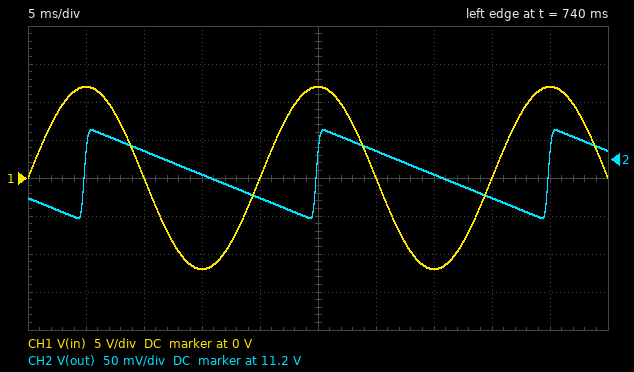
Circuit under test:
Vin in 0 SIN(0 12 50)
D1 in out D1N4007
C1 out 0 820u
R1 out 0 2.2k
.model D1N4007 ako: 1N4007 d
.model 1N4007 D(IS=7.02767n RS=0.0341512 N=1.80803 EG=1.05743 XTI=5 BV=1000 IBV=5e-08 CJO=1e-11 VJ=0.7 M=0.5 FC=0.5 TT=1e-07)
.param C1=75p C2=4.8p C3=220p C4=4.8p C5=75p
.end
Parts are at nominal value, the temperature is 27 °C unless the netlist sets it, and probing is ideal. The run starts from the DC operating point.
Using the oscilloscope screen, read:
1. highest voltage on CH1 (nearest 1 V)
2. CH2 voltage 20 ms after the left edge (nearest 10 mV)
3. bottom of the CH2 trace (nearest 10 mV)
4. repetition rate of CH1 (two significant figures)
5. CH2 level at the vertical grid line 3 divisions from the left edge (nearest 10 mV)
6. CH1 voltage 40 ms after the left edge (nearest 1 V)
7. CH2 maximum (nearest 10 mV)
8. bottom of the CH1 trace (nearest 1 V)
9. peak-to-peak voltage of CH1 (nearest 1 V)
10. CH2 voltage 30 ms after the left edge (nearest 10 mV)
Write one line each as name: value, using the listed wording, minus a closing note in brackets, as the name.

highest voltage on CH1: 12 V
CH2 voltage 20 ms after the left edge: 11.15 V
bottom of the CH2 trace: 11.12 V
repetition rate of CH1: 50 Hz
CH2 level at the vertical grid line 3 divisions from the left edge: 11.18 V
CH1 voltage 40 ms after the left edge: 0 V
CH2 maximum: 11.24 V
bottom of the CH1 trace: -12 V
peak-to-peak voltage of CH1: 24 V
CH2 voltage 30 ms after the left edge: 11.21 V
